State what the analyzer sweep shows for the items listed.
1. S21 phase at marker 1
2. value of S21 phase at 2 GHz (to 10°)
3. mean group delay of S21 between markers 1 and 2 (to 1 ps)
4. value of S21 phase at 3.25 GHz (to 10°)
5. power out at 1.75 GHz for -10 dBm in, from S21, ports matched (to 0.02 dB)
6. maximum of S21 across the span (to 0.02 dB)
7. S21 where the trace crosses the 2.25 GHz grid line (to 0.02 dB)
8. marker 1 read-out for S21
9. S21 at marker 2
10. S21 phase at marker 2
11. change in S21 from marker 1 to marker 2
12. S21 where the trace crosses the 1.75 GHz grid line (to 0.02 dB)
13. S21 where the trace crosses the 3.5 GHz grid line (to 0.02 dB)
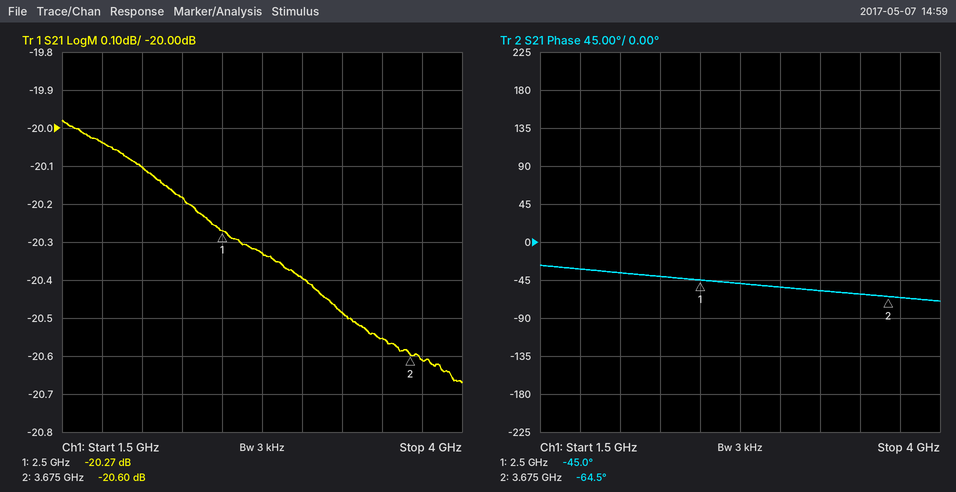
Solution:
-45.0°
-40°
46 ps
-60°
-30.04 dBm
-19.98 dB
-20.18 dB
-20.27 dB
-20.60 dB
-64.5°
-0.33 dB
-20.04 dB
-20.56 dB
